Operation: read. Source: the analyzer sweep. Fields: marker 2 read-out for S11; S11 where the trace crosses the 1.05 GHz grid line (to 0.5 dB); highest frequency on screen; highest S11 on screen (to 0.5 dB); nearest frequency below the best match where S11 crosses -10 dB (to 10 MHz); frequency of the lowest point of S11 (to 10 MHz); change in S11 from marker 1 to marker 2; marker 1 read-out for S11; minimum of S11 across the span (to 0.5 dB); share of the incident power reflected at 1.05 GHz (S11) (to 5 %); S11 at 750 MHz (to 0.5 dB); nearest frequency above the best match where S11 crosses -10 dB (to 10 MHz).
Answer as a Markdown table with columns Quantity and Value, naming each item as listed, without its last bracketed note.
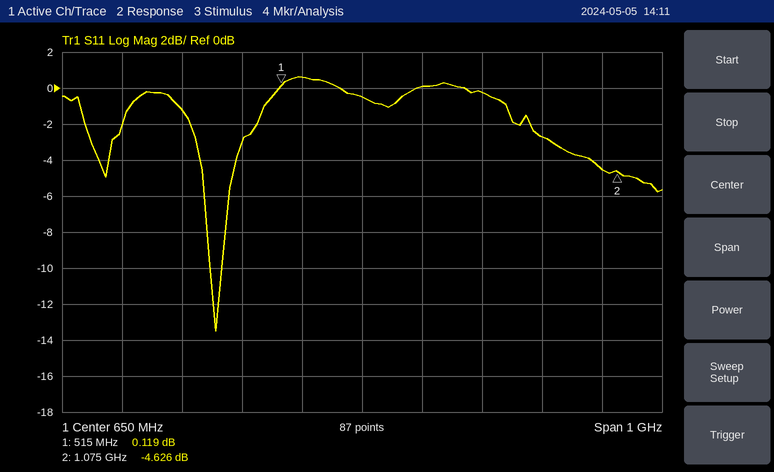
| Quantity | Value |
|---|---|
| marker 2 read-out for S11 | -4.626 dB |
| S11 where the trace crosses the 1.05 GHz grid line | -4.5 dB |
| highest frequency on screen | 1.15 GHz |
| highest S11 on screen | 0.5 dB |
| nearest frequency below the best match where S11 crosses -10 dB | 400 MHz |
| frequency of the lowest point of S11 | 410 MHz |
| change in S11 from marker 1 to marker 2 | -4.745 dB |
| marker 1 read-out for S11 | 0.119 dB |
| minimum of S11 across the span | -13.5 dB |
| share of the incident power reflected at 1.05 GHz (S11) | 35 % |
| S11 at 750 MHz | 0.0 dB |
| nearest frequency above the best match where S11 crosses -10 dB | 420 MHz |
